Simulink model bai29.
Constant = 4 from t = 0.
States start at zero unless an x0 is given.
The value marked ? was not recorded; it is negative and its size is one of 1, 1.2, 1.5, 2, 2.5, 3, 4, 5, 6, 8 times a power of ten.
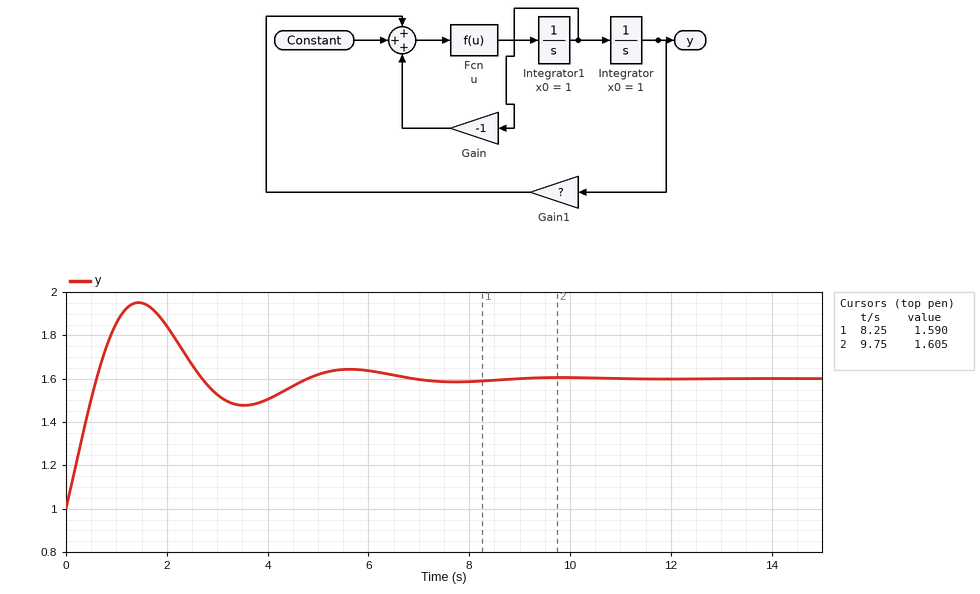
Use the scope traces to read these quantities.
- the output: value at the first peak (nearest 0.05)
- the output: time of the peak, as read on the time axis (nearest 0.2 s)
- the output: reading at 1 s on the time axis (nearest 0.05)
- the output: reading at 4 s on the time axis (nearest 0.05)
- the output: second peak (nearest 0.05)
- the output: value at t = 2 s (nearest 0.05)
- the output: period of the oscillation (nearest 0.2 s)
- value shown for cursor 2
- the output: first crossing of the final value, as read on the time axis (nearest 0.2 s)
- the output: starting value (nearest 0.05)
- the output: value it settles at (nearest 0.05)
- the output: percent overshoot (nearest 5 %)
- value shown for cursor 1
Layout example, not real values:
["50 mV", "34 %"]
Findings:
["1.95", "1.4 s", "1.85", "1.50", "1.65", "1.85", "4.2 s", "1.605", "0.6 s", "1.00", "1.60", "60 %", "1.590"]
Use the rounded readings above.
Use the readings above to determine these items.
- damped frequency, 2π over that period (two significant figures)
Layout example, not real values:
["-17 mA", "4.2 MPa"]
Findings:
["1.5 rad/s"]
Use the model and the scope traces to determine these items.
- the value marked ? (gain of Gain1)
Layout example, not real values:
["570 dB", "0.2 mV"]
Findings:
["-2.5"]
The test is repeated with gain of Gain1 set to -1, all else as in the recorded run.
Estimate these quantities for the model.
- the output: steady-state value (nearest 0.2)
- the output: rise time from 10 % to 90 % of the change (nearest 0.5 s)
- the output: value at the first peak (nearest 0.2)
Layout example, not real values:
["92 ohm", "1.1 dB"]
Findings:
["4.0", "1.5 s", "4.6"]
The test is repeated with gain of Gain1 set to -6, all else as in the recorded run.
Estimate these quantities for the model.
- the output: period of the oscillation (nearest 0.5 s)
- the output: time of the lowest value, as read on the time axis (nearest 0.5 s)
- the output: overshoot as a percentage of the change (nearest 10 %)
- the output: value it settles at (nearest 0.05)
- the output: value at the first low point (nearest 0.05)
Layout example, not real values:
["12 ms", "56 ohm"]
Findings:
["2.5 s", "1.5 s", "80 %", "0.65", "0.40"]
